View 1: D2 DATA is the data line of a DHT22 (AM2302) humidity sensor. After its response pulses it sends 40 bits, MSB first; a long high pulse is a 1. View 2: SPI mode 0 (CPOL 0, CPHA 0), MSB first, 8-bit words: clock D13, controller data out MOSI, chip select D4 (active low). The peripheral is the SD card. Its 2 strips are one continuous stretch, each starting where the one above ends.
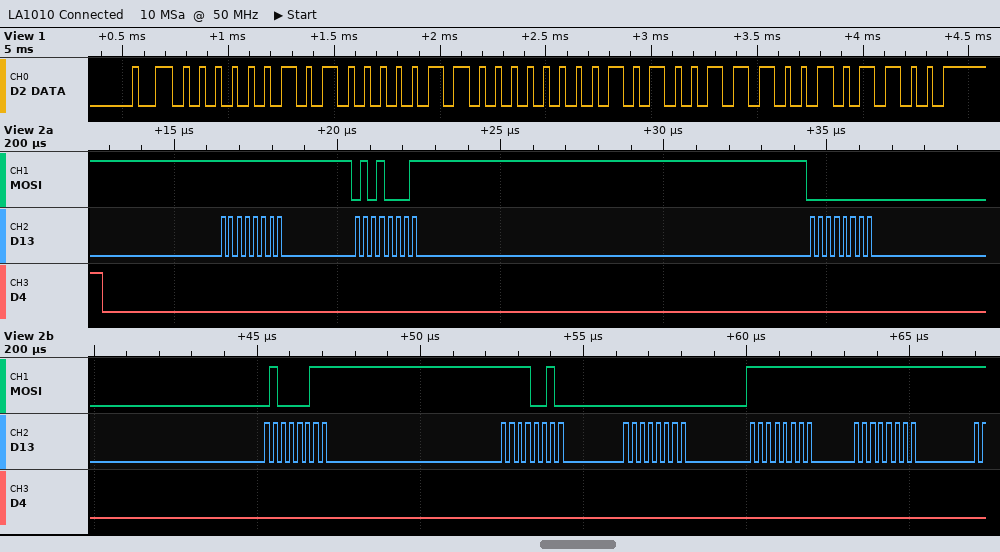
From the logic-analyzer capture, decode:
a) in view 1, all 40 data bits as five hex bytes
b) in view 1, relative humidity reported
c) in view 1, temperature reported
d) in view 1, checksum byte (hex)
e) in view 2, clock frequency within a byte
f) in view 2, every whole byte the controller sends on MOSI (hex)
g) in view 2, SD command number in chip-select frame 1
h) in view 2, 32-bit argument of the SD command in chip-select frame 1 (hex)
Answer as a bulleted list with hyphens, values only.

- 02 83 00 A7 2C
- 64.3 %
- 16.7 °C
- 0x2C
- 4 MHz
- FF 51 00 43 F2 00 FF FF
- CMD17
- 0x0043F200
